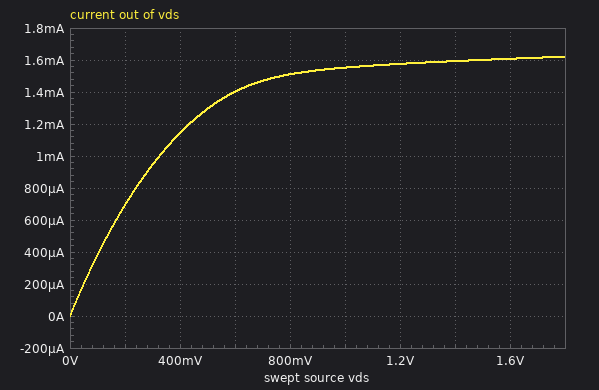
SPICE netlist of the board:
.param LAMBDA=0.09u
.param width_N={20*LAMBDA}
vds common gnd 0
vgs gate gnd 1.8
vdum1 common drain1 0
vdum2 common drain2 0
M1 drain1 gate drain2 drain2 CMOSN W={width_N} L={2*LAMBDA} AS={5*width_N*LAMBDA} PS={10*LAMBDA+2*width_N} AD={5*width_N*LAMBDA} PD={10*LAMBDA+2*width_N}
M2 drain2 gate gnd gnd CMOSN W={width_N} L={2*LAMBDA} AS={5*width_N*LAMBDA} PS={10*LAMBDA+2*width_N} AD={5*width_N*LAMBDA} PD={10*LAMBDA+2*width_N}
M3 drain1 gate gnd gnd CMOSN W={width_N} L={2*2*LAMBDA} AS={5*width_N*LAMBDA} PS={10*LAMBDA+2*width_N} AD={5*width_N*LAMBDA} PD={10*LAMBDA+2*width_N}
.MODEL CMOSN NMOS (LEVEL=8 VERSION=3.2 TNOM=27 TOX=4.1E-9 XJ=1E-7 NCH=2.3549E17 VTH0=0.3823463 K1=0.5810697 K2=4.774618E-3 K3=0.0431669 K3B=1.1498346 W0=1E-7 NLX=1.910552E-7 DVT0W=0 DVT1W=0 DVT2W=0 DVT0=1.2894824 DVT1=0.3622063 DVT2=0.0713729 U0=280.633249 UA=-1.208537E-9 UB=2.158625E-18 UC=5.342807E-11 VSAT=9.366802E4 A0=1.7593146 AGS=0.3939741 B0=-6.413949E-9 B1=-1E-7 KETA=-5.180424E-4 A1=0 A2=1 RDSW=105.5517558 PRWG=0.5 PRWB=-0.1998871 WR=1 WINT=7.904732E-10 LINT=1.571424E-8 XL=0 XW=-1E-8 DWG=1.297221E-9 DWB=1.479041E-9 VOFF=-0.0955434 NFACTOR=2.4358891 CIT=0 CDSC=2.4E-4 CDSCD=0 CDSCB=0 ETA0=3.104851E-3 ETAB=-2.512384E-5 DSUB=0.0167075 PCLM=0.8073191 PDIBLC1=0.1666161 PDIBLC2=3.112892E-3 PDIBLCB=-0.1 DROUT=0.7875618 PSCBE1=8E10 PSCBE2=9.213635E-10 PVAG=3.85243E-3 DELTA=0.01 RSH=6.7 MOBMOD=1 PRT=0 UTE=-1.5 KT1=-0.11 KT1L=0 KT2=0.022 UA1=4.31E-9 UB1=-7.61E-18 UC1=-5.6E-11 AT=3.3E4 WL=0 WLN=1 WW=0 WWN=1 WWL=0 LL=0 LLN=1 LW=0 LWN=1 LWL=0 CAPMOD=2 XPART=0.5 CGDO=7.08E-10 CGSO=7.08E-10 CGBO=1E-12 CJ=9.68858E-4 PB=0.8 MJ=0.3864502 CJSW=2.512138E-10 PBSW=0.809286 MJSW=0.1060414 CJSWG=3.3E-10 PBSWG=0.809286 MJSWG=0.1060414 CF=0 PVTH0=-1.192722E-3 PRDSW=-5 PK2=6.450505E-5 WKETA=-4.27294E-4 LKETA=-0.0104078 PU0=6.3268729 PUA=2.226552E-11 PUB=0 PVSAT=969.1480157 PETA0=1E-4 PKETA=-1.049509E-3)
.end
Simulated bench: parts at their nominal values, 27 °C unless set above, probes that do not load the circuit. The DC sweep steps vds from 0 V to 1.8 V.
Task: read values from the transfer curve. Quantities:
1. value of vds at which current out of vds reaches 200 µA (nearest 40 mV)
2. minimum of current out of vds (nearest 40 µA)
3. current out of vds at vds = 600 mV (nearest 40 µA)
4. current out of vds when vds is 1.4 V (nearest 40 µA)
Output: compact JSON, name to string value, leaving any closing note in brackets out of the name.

{"value of vds at which current out of vds reaches 200 µA": "40 mV", "minimum of current out of vds": "0 A", "current out of vds at vds = 600 mV": "1.40 mA", "current out of vds when vds is 1.4 V": "1.60 mA"}
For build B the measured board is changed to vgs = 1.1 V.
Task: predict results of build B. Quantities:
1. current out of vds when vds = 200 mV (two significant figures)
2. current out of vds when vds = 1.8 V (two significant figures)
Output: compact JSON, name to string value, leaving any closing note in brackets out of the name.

{"current out of vds when vds = 200 mV": "360 µA", "current out of vds when vds = 1.8 V": "590 µA"}
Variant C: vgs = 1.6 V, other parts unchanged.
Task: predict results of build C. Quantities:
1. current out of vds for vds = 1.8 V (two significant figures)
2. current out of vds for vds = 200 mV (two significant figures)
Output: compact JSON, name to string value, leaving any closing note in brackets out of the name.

{"current out of vds for vds = 1.8 V": "1.3 mA", "current out of vds for vds = 200 mV": "620 µA"}
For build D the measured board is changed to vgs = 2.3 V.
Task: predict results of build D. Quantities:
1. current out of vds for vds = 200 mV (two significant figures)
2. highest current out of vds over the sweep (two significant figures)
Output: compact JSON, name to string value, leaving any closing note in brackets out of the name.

{"current out of vds for vds = 200 mV": "800 µA", "highest current out of vds over the sweep": "2.3 mA"}
